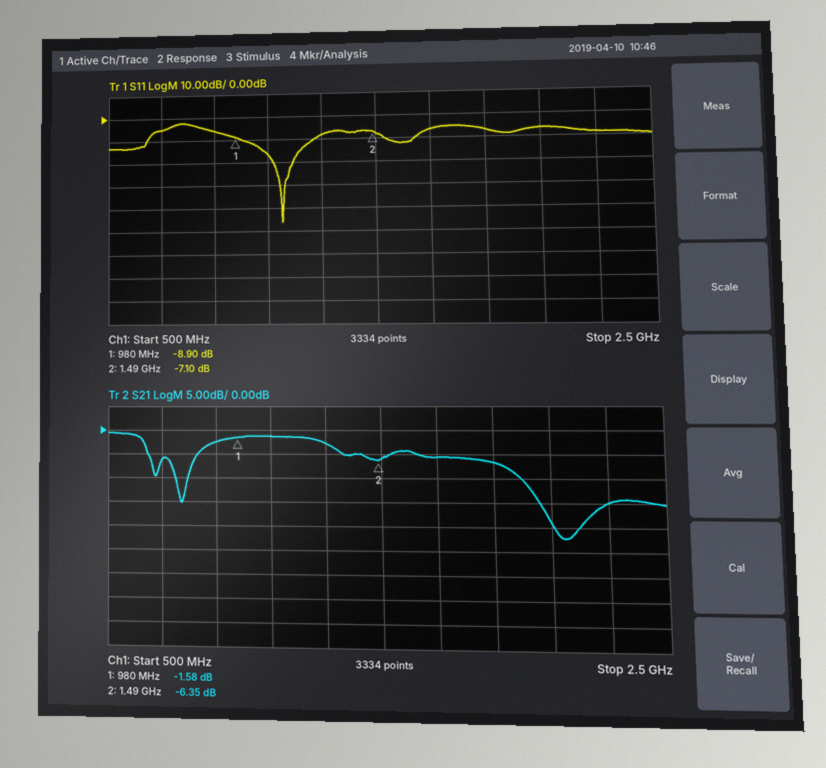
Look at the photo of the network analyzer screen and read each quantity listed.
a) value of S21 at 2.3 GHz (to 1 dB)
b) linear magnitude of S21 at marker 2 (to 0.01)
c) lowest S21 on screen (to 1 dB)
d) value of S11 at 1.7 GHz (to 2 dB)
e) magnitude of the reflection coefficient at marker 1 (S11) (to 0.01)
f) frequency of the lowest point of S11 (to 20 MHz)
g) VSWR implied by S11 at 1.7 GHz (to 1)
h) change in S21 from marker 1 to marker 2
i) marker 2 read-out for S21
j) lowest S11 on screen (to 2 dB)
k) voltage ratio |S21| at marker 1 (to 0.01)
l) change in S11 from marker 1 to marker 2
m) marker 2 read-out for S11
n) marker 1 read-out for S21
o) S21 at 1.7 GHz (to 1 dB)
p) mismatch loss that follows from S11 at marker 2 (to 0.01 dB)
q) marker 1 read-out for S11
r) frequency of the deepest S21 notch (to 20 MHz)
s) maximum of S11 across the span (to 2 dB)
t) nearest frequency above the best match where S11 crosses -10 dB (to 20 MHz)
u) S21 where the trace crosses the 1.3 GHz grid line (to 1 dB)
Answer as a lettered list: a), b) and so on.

a) -15 dB
b) 0.48
c) -22 dB
d) -6 dB
e) 0.36
f) 1.16 GHz
g) 3
h) -4.77 dB
i) -6.35 dB
j) -46 dB
k) 0.83
l) 1.80 dB
m) -7.10 dB
n) -1.58 dB
o) -6 dB
p) 0.94 dB
q) -8.90 dB
r) 2.14 GHz
s) -2 dB
t) 1.28 GHz
u) -3 dB
